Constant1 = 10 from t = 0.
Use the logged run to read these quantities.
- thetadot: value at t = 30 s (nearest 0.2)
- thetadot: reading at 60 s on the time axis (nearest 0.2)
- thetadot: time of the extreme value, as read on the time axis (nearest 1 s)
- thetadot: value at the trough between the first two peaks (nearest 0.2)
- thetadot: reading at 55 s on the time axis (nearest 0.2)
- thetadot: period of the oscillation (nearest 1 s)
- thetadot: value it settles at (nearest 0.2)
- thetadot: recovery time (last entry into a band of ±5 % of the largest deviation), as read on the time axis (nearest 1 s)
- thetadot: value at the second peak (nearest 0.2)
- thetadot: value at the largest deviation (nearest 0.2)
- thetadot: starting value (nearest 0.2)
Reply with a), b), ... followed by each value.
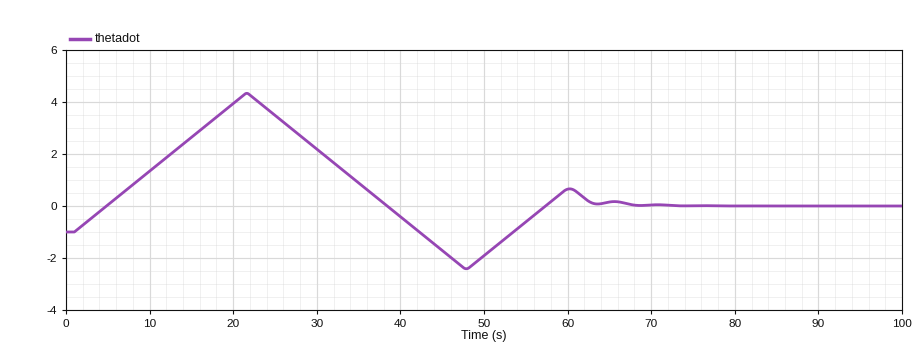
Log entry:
a) 2.2
b) 0.6
c) 22 s
d) -2.4
e) -0.6
f) 39 s
g) 0.0
h) 62 s
i) 0.6
j) 4.4
k) -1.0
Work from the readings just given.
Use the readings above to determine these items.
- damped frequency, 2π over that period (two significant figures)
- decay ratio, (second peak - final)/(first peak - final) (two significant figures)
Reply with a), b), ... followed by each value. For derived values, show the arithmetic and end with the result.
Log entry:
a) 2π / 39 = 0.16 rad/s
b) (0.6 - 0) / (4.4 - 0) = 0.14
